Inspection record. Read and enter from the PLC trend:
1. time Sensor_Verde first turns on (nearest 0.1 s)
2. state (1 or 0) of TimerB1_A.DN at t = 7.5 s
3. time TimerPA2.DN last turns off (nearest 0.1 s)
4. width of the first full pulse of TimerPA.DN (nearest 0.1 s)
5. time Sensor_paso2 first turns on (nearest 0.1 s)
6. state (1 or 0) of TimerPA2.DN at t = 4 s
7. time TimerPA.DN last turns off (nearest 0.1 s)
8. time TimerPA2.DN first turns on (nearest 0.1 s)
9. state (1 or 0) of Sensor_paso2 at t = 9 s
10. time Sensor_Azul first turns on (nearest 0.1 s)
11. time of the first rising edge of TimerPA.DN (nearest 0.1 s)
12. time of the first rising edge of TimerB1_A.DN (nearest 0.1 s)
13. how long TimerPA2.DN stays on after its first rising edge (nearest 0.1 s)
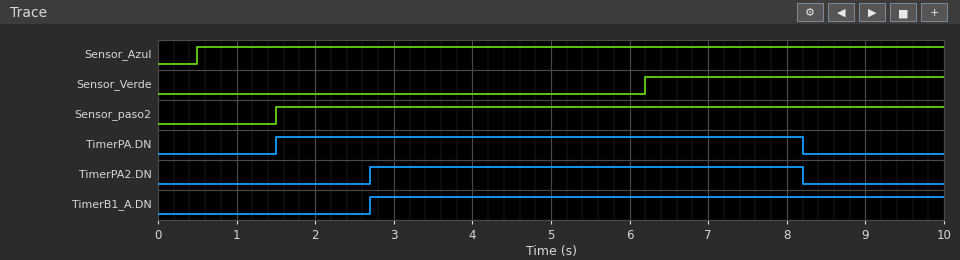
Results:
6.2 s
1
8.2 s
6.7 s
1.5 s
1
8.2 s
2.7 s
1
0.5 s
1.5 s
2.7 s
5.5 s
